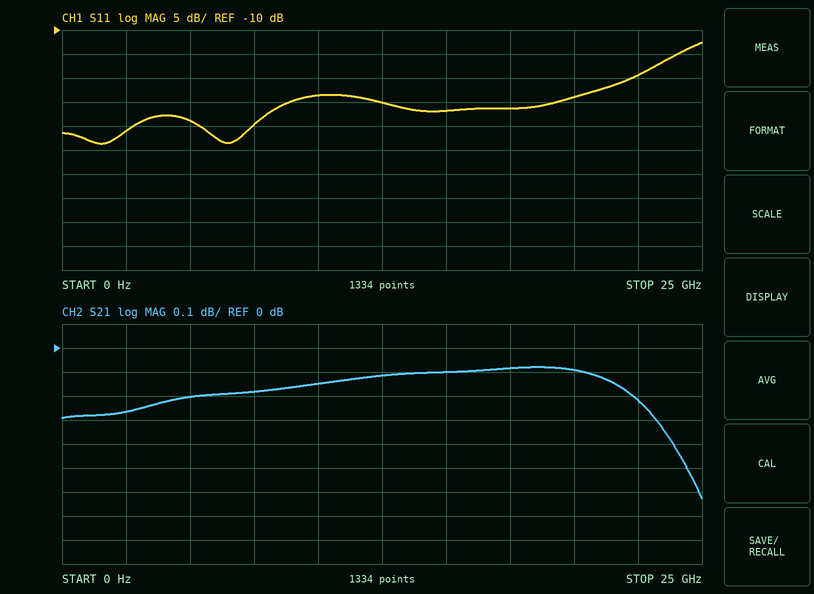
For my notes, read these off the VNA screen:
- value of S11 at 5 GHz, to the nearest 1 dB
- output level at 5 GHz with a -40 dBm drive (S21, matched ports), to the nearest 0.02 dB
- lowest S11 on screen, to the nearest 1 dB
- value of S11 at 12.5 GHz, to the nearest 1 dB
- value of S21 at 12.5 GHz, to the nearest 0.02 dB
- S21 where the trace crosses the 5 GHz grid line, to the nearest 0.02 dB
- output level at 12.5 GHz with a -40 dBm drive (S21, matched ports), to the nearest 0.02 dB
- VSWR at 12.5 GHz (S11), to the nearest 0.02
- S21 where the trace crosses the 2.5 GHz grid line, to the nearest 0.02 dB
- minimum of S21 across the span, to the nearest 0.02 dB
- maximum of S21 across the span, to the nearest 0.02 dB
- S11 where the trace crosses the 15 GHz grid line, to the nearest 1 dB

-29 dB
-40.20 dBm
-34 dB
-25 dB
-0.12 dB
-0.20 dB
-40.12 dBm
1.12
-0.26 dB
-0.62 dB
-0.08 dB
-27 dB
